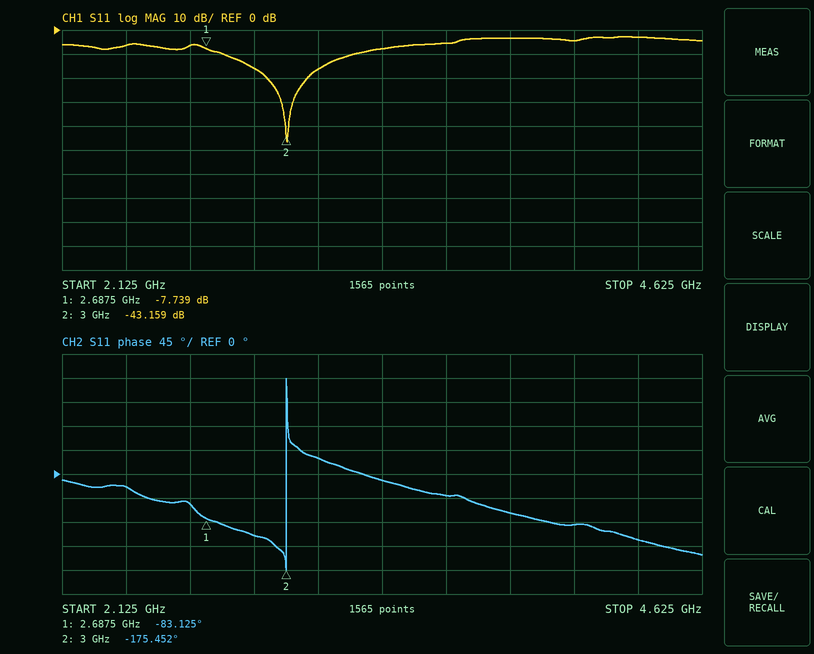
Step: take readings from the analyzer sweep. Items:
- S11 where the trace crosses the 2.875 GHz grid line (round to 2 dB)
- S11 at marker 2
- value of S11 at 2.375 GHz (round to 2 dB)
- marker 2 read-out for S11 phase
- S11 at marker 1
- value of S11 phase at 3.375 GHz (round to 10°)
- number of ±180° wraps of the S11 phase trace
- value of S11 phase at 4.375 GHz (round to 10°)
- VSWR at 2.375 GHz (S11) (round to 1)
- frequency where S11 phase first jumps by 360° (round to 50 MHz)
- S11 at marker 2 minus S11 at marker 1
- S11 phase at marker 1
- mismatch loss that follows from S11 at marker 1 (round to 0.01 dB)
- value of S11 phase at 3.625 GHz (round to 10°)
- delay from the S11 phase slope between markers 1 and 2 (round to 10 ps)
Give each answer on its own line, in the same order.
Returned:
-16 dB
-43.159 dB
-6 dB
-175.452°
-7.739 dB
-10°
1
-120°
3
3.00 GHz
-35.420 dB
-83.125°
0.80 dB
-40°
820 ps
